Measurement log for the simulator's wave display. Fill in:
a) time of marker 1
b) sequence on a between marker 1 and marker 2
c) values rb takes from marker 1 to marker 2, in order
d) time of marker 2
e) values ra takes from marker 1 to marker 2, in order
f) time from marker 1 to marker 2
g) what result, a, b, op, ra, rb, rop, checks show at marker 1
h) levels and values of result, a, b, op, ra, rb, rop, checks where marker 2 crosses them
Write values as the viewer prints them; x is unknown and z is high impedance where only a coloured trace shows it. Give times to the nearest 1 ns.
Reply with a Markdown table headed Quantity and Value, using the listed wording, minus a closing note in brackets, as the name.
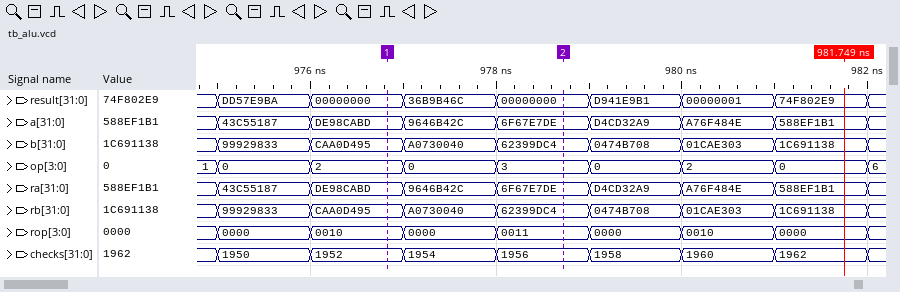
| Quantity | Value |
|---|---|
| time of marker 1 | 977 ns |
| sequence on a between marker 1 and marker 2 | DE98CABD, 9646B42C, 6F67E7DE |
| values rb takes from marker 1 to marker 2, in order | CAA0D495, A0730040, 62399DC4 |
| time of marker 2 | 979 ns |
| values ra takes from marker 1 to marker 2, in order | DE98CABD, 9646B42C, 6F67E7DE |
| time from marker 1 to marker 2 | 2 ns |
| what result, a, b, op, ra, rb, rop, checks show at marker 1 | result=00000000, a=DE98CABD, b=CAA0D495, op=2, ra=DE98CABD, rb=CAA0D495, rop=0010, checks=1952 |
| levels and values of result, a, b, op, ra, rb, rop, checks where marker 2 crosses them | result=00000000, a=6F67E7DE, b=62399DC4, op=3, ra=6F67E7DE, rb=62399DC4, rop=0011, checks=1956 |
